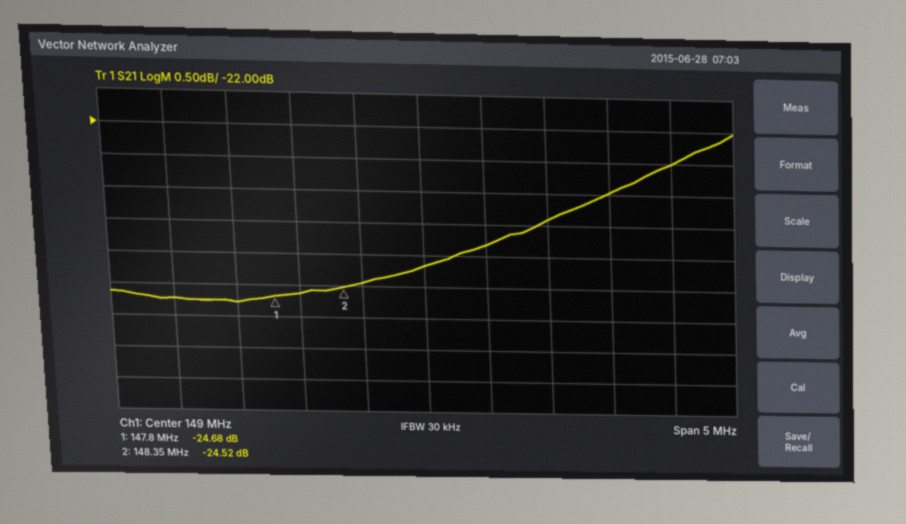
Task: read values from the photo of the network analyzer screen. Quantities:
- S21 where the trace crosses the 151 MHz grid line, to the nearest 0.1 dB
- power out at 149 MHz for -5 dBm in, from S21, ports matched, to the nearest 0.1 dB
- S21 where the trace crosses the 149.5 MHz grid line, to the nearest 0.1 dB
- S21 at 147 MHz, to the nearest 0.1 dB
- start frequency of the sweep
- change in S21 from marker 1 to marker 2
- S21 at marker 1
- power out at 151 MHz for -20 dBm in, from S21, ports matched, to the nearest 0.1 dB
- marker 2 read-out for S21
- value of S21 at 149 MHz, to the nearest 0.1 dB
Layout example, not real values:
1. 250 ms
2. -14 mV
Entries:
1. -22.5 dB
2. -29.2 dBm
3. -23.8 dB
4. -24.7 dB
5. 146.5 MHz
6. 0.16 dB
7. -24.68 dB
8. -42.5 dBm
9. -24.52 dB
10. -24.2 dB
